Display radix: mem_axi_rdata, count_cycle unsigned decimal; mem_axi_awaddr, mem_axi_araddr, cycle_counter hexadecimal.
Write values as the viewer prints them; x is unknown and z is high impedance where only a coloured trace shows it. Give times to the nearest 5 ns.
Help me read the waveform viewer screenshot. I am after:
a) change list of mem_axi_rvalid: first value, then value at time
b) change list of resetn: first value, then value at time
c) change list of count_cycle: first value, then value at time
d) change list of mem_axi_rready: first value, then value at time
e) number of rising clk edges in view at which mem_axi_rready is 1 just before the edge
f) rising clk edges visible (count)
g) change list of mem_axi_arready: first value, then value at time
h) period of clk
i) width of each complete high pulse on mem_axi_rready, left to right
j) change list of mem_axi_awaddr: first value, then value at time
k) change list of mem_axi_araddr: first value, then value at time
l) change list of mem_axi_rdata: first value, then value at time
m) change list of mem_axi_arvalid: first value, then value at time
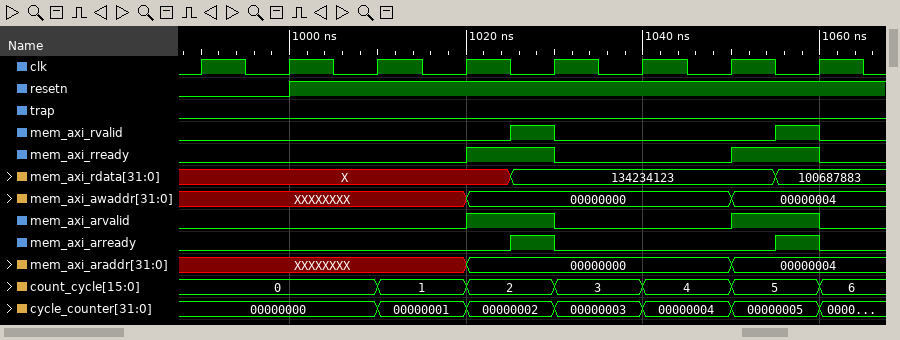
0, 1 at 1025 ns, 0 at 1030 ns, 1 at 1055 ns, 0 at 1060 ns
0, 1 at 1000 ns
0, 1 at 1010 ns, 2 at 1020 ns, 3 at 1030 ns, 4 at 1040 ns, 5 at 1050 ns, 6 at 1060 ns
0, 1 at 1020 ns, 0 at 1030 ns, 1 at 1050 ns, 0 at 1060 ns
2
8
0, 1 at 1025 ns, 0 at 1030 ns, 1 at 1055 ns, 0 at 1060 ns
10 ns
10 ns, 10 ns
XXXXXXXX, 00000000 at 1020 ns, 00000004 at 1050 ns
XXXXXXXX, 00000000 at 1020 ns, 00000004 at 1050 ns
X, 134234123 at 1025 ns, 100687883 at 1055 ns
0, 1 at 1020 ns, 0 at 1030 ns, 1 at 1050 ns, 0 at 1060 ns
